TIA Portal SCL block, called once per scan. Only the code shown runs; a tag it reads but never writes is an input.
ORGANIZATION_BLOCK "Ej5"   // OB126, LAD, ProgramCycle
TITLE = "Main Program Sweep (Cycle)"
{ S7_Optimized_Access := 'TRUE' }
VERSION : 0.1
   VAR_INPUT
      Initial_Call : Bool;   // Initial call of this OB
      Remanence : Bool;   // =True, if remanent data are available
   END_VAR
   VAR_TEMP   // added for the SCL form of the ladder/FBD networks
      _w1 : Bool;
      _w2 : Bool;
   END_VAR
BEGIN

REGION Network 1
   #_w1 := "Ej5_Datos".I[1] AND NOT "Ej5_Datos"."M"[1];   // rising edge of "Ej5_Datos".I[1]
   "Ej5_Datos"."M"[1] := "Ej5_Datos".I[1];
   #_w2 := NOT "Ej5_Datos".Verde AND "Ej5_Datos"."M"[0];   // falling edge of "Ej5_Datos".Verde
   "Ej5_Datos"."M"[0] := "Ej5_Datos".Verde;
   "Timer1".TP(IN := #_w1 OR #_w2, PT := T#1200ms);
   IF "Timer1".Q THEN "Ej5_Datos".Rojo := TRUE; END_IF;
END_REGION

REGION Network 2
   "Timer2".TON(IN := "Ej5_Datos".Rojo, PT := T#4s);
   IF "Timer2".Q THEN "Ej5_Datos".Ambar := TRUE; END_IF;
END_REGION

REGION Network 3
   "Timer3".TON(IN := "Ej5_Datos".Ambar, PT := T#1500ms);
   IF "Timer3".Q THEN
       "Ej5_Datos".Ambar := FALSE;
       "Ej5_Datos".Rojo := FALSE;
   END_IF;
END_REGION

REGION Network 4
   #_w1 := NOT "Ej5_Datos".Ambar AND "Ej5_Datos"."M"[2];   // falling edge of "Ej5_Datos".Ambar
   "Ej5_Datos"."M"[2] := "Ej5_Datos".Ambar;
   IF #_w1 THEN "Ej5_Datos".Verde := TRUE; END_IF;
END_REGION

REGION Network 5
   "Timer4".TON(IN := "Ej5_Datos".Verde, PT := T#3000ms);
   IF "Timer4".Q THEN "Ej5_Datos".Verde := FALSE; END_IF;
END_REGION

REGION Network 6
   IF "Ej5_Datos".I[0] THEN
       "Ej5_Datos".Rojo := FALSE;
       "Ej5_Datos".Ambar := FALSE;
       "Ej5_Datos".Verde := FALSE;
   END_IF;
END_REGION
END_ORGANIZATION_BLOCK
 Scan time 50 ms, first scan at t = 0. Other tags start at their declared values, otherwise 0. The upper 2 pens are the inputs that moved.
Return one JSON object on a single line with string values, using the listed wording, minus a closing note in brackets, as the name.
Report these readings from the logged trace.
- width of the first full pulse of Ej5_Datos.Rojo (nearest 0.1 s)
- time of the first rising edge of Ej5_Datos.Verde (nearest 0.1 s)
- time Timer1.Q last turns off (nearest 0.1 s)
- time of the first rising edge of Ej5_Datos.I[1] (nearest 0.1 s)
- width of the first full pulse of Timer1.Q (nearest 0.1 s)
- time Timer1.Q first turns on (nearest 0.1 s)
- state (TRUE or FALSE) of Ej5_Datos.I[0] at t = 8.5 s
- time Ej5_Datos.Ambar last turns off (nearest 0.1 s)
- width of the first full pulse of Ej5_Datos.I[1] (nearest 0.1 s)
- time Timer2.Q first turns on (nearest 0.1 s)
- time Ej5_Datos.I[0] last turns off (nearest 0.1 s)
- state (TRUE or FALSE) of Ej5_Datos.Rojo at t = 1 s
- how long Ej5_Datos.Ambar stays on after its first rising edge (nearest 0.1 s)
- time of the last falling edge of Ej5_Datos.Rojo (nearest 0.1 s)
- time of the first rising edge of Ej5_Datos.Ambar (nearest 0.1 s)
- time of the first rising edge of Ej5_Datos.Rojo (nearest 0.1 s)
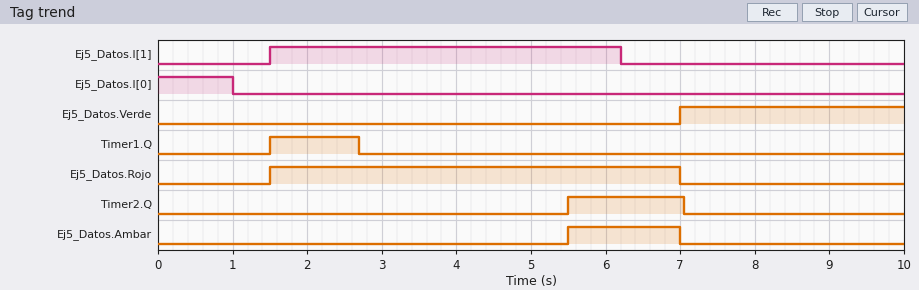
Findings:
{"width of the first full pulse of Ej5_Datos.Rojo": "5.5 s", "time of the first rising edge of Ej5_Datos.Verde": "7.0 s", "time Timer1.Q last turns off": "2.7 s", "time of the first rising edge of Ej5_Datos.I[1]": "1.5 s", "width of the first full pulse of Timer1.Q": "1.2 s", "time Timer1.Q first turns on": "1.5 s", "state (TRUE or FALSE) of Ej5_Datos.I[0] at t = 8.5 s": "FALSE", "time Ej5_Datos.Ambar last turns off": "7.0 s", "width of the first full pulse of Ej5_Datos.I[1]": "4.7 s", "time Timer2.Q first turns on": "5.5 s", "time Ej5_Datos.I[0] last turns off": "1.0 s", "state (TRUE or FALSE) of Ej5_Datos.Rojo at t = 1 s": "FALSE", "how long Ej5_Datos.Ambar stays on after its first rising edge": "1.5 s", "time of the last falling edge of Ej5_Datos.Rojo": "7.0 s", "time of the first rising edge of Ej5_Datos.Ambar": "5.5 s", "time of the first rising edge of Ej5_Datos.Rojo": "1.5 s"}
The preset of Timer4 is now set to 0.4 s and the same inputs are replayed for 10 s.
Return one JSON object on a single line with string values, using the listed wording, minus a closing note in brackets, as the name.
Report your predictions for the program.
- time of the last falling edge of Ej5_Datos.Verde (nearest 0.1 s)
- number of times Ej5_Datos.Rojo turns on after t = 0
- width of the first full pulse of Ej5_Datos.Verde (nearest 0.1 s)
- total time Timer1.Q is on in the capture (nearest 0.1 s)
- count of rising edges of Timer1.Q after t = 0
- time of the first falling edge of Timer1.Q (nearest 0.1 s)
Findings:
{"time of the last falling edge of Ej5_Datos.Verde": "7.4 s", "number of times Ej5_Datos.Rojo turns on after t = 0": "2", "width of the first full pulse of Ej5_Datos.Verde": "0.4 s", "total time Timer1.Q is on in the capture": "2.4 s", "count of rising edges of Timer1.Q after t = 0": "2", "time of the first falling edge of Timer1.Q": "2.7 s"}
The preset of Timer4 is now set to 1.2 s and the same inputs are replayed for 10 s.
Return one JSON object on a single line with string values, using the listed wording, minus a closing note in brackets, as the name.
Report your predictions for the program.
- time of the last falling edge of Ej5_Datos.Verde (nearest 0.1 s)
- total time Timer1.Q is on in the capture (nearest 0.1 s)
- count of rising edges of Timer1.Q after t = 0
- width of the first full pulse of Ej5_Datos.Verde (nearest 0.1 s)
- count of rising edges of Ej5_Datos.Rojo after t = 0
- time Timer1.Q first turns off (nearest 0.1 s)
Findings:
{"time of the last falling edge of Ej5_Datos.Verde": "8.2 s", "total time Timer1.Q is on in the capture": "2.4 s", "count of rising edges of Timer1.Q after t = 0": "2", "width of the first full pulse of Ej5_Datos.Verde": "1.2 s", "count of rising edges of Ej5_Datos.Rojo after t = 0": "2", "time Timer1.Q first turns off": "2.7 s"}
